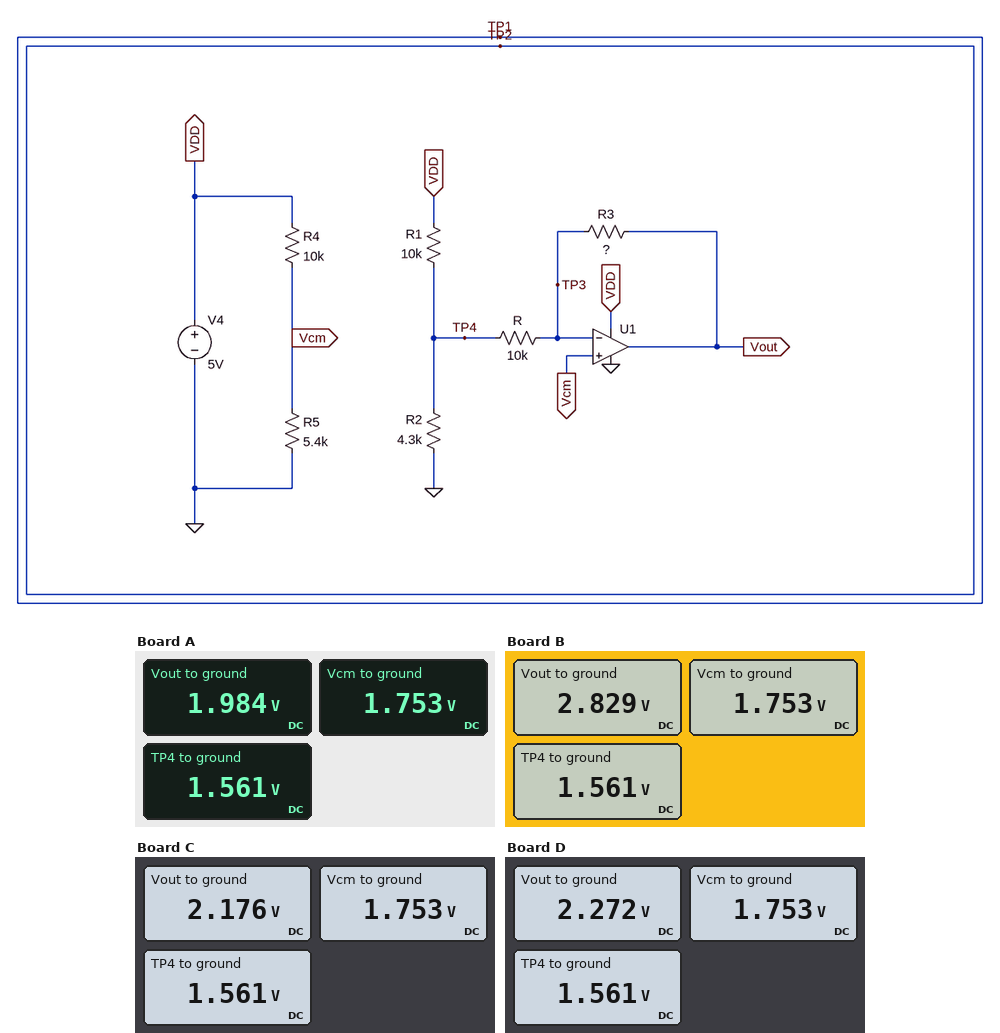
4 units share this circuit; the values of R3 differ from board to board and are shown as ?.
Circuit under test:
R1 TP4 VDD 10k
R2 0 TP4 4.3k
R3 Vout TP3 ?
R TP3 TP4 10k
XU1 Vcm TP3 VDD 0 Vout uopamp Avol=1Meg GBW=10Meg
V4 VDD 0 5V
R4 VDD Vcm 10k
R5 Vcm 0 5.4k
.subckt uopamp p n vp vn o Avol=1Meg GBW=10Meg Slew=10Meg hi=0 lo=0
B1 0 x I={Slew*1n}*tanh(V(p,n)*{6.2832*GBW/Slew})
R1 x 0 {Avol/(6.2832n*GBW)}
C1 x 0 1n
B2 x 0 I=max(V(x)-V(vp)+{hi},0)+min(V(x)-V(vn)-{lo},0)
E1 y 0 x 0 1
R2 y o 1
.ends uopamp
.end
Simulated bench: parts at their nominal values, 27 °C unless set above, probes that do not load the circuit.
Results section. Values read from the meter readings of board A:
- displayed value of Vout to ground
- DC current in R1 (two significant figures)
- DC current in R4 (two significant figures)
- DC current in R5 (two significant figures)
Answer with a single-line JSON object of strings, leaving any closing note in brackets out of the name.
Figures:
{"displayed value of Vout to ground": "1.984 V", "DC current in R1": "340 µA", "DC current in R4": "320 µA", "DC current in R5": "320 µA"}
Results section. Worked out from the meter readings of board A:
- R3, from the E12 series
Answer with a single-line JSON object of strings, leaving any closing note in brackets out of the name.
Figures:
{"R3, from the E12 series": "12 kΩ"}
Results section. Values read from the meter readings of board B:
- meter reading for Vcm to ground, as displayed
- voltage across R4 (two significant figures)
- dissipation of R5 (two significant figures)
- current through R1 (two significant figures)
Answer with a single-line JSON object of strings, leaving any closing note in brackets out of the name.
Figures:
{"meter reading for Vcm to ground, as displayed": "1.753 V", "voltage across R4": "3.2 V", "dissipation of R5": "570 µW", "current through R1": "340 µA"}
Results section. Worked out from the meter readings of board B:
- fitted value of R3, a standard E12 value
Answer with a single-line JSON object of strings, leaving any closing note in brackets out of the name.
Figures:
{"fitted value of R3, a standard E12 value": "56 kΩ"}
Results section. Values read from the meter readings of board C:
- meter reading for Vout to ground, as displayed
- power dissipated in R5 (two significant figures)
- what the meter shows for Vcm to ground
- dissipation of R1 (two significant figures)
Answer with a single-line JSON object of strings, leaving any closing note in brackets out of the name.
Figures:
{"meter reading for Vout to ground, as displayed": "2.176 V", "power dissipated in R5": "570 µW", "what the meter shows for Vcm to ground": "1.753 V", "dissipation of R1": "1.2 mW"}
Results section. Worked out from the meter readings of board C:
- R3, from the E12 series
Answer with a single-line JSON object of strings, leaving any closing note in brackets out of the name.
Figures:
{"R3, from the E12 series": "22 kΩ"}
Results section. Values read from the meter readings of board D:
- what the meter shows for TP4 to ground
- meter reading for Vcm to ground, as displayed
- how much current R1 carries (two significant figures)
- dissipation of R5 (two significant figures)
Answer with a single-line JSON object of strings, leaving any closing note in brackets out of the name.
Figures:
{"what the meter shows for TP4 to ground": "1.561 V", "meter reading for Vcm to ground, as displayed": "1.753 V", "how much current R1 carries": "340 µA", "dissipation of R5": "570 µW"}
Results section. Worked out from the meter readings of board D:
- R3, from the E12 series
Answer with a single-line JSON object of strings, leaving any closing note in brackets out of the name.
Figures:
{"R3, from the E12 series": "27 kΩ"}
